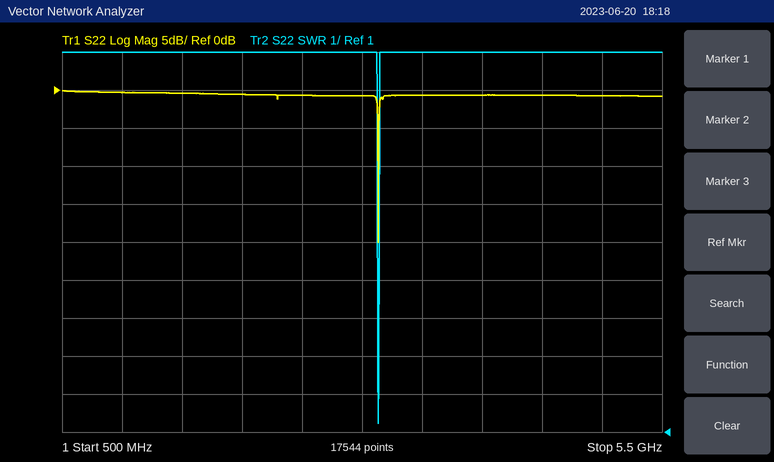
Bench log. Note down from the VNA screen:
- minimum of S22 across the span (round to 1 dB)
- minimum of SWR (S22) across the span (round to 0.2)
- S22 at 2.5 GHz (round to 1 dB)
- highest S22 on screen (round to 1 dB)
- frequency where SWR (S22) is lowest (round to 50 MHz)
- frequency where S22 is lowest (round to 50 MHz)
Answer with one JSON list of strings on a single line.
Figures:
["-20 dB", "1.2", "-1 dB", "0 dB", "3.15 GHz", "3.15 GHz"]
